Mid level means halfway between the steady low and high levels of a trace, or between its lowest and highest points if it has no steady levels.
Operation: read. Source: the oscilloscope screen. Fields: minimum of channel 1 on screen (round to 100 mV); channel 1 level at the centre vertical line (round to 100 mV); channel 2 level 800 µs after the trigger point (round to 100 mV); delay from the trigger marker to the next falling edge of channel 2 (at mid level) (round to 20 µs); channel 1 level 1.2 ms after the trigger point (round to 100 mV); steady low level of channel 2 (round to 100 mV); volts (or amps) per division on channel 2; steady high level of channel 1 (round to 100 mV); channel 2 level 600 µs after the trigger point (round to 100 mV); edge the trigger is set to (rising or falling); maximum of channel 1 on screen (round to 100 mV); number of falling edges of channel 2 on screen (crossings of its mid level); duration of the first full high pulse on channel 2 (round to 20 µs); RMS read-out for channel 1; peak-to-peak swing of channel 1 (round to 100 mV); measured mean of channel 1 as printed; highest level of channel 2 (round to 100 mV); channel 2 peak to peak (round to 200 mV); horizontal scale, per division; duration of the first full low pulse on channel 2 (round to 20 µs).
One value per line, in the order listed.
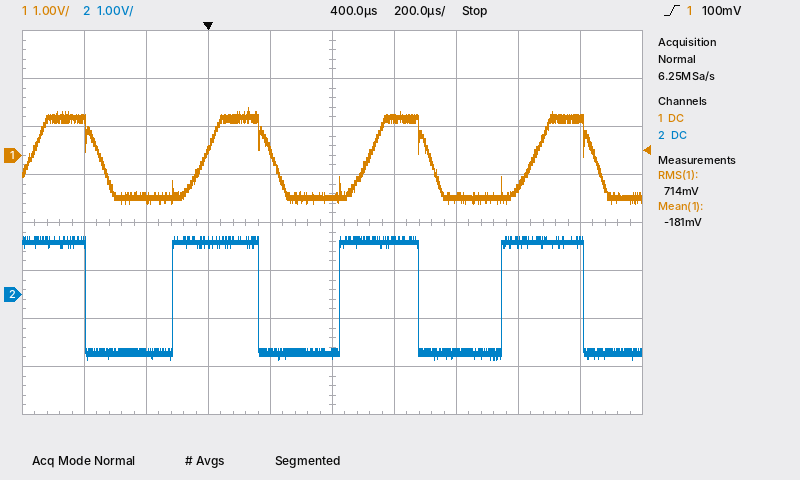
-1.0 V
-900 mV
-1.2 V
160 µs
800 mV
-1.2 V
1 V
800 mV
1.1 V
rising
1.0 V
4
280 µs
714 mV
2.0 V
-181 mV
1.2 V
2.6 V
200 µs
280 µs
